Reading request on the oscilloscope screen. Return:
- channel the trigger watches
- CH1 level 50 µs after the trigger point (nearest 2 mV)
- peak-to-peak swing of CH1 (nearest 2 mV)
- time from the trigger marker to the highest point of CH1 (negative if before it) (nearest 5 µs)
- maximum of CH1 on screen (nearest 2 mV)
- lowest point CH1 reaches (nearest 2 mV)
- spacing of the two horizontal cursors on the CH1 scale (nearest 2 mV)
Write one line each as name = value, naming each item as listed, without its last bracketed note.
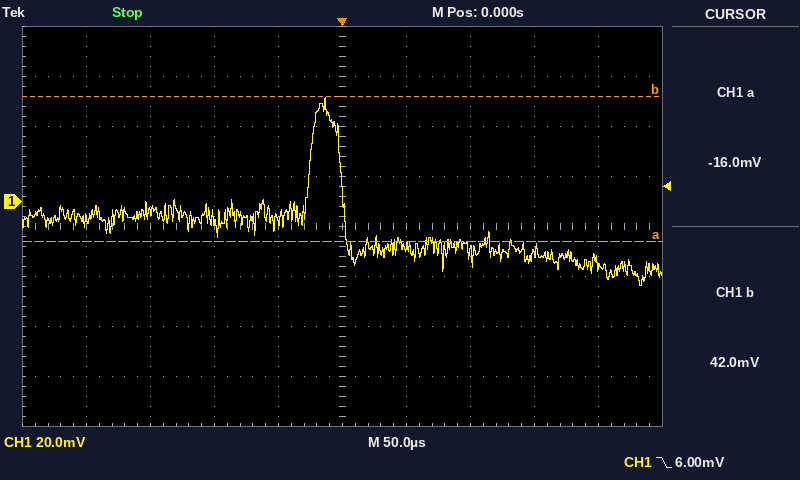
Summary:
channel the trigger watches = CH1
CH1 level 50 µs after the trigger point = -18 mV
peak-to-peak swing of CH1 = 76 mV
time from the trigger marker to the highest point of CH1 (negative if before it) = -15 µs
maximum of CH1 on screen = 42 mV
lowest point CH1 reaches = -34 mV
spacing of the two horizontal cursors on the CH1 scale = 58 mV
